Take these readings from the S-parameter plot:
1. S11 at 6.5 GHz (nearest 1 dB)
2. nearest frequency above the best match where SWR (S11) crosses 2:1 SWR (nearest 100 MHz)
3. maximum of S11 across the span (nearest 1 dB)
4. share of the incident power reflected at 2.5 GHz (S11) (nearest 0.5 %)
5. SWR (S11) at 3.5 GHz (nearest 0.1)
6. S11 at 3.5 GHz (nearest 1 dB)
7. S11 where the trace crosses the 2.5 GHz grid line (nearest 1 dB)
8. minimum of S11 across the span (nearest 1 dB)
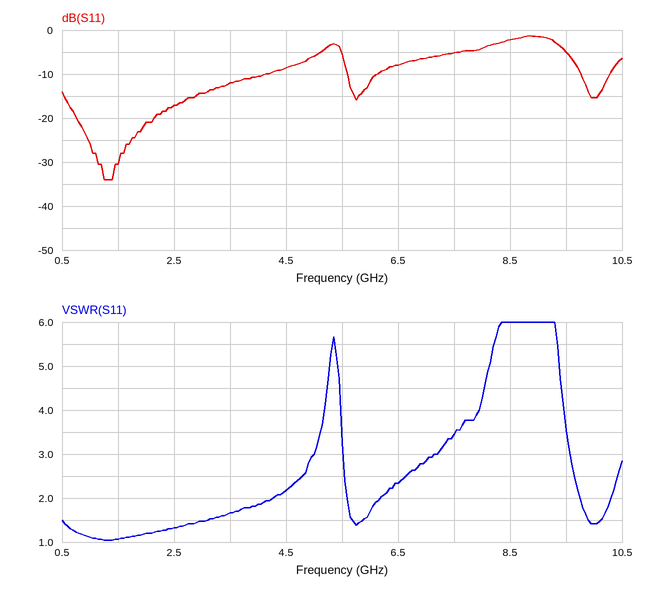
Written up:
-8 dB
4.3 GHz
-1 dB
2.0 %
1.7
-12 dB
-17 dB
-34 dB
